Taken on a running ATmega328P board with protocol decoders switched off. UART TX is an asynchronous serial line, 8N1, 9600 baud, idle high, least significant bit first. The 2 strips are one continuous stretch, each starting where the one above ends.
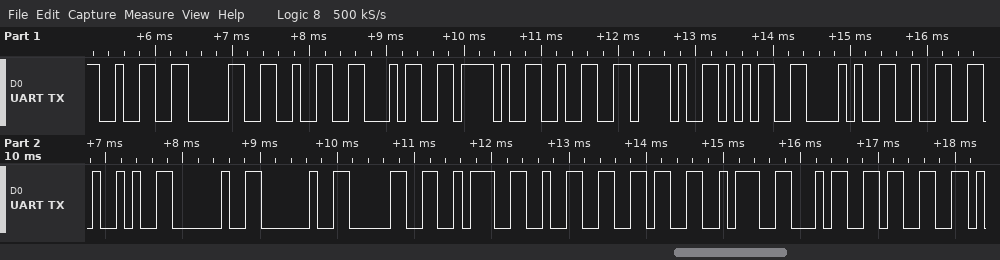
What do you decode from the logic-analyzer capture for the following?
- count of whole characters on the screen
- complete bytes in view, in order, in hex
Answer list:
20
0x32 0x30 0x32 0x34 0x2F 0x32 0x2F 0x35 0x28 0x32 0x29 0x20 0x20 0x30 0x3A 0x32 0x36 0x3A 0x34 0x33
